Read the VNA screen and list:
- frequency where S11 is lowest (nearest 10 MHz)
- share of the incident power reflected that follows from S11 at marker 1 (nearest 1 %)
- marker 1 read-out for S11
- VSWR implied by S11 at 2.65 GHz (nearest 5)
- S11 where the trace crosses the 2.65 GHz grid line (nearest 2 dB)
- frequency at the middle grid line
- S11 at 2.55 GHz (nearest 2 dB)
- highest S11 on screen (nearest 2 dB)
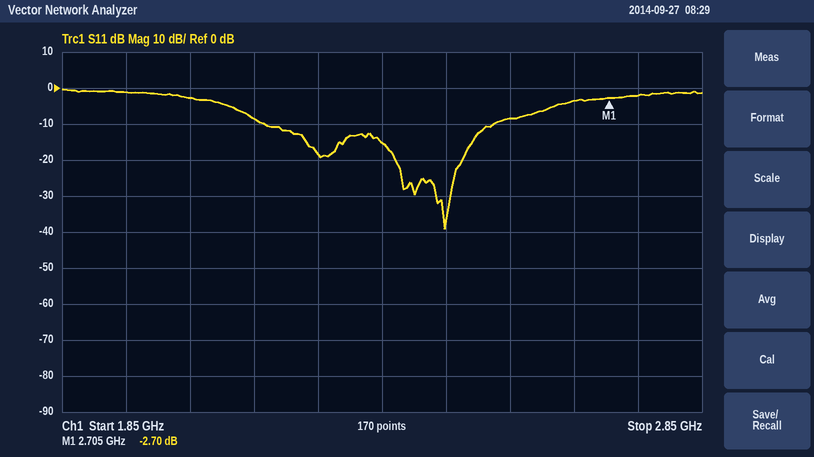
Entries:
2.45 GHz
54 %
-2.70 dB
5
-4 dB
2.35 GHz
-8 dB
0 dB
